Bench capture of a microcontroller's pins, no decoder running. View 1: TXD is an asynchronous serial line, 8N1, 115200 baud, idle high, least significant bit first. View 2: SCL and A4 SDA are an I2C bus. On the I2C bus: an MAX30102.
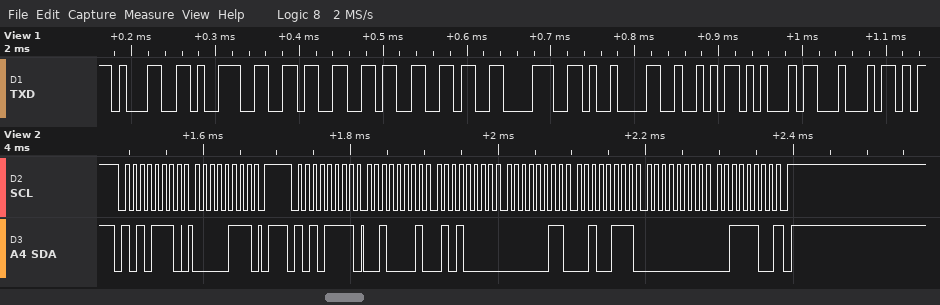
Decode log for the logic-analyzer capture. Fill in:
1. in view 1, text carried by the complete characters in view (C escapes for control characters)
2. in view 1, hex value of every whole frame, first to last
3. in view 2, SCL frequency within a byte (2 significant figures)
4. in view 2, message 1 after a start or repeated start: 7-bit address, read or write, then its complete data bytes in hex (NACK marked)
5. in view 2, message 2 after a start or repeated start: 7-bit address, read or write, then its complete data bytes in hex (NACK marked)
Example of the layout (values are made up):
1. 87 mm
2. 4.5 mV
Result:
1. "196668\tRED"
2. 31 39 36 36 36 38 09 52 45 44
3. 100 kHz
4. 0x57 write: 07
5. 0x57 read: 21 50 03 27 00 3C NACK
